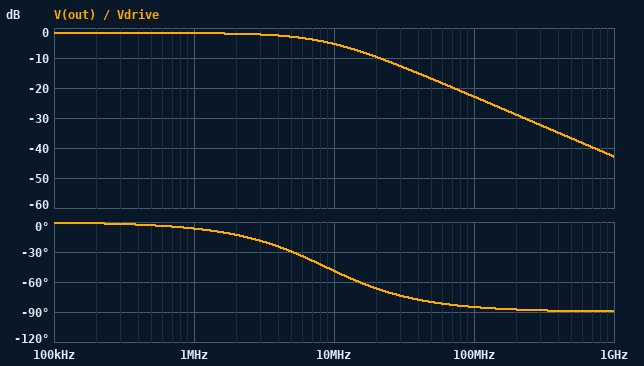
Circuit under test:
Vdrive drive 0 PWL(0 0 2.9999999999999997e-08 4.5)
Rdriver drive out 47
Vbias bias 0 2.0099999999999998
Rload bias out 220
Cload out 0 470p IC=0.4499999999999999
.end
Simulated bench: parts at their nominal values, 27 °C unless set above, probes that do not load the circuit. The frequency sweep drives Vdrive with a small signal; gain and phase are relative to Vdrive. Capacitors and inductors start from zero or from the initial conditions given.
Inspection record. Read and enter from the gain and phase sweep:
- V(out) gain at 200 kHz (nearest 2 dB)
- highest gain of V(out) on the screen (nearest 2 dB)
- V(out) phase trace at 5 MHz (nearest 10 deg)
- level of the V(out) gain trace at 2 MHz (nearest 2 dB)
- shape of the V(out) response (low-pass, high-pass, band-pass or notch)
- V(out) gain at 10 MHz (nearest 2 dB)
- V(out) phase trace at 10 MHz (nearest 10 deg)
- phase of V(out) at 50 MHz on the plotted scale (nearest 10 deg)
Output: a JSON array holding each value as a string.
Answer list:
["-2 dB", "-2 dB", "-30 deg", "-2 dB", "low-pass", "-6 dB", "-50 deg", "-80 deg"]
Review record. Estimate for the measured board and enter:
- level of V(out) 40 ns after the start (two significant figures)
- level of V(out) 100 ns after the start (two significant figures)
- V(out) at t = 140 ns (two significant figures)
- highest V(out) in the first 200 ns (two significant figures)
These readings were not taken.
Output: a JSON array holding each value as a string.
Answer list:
["3.0 V", "4.0 V", "4.1 V", "4.1 V"]
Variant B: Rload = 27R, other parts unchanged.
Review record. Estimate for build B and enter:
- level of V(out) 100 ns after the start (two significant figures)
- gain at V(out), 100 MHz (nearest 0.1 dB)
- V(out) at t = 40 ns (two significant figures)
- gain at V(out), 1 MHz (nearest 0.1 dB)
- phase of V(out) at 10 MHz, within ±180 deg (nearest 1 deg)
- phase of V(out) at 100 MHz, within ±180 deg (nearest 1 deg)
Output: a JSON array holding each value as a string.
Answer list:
["2.9 V", "-23.0 dB", "2.8 V", "-8.8 dB", "-27 deg", "-79 deg"]
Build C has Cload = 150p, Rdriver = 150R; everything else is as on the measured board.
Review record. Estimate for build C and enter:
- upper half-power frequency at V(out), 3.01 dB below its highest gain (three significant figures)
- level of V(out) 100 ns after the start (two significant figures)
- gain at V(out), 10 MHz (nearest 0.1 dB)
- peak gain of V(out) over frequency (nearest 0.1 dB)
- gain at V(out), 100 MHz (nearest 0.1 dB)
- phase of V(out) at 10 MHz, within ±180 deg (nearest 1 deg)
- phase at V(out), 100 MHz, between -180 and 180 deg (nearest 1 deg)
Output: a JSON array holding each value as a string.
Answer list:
["11.9 MHz", "3.5 V", "-6.8 dB", "-4.5 dB", "-23.1 dB", "-40 deg", "-83 deg"]
